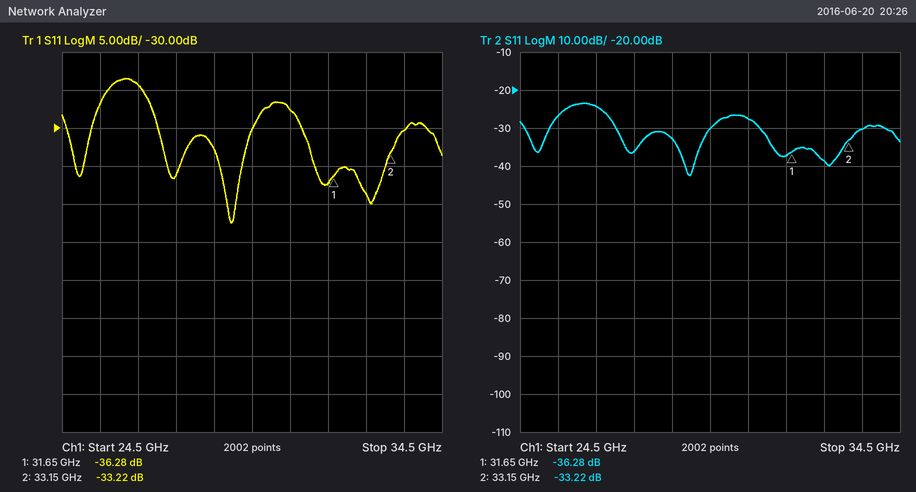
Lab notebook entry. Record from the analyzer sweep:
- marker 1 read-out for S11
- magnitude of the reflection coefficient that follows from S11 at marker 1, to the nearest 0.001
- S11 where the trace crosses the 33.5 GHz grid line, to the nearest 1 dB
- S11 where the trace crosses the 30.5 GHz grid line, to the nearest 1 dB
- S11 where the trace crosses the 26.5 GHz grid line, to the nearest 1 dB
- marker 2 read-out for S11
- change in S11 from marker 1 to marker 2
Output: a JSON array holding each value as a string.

["-36.28 dB", "0.015", "-30 dB", "-28 dB", "-24 dB", "-33.22 dB", "3.06 dB"]
